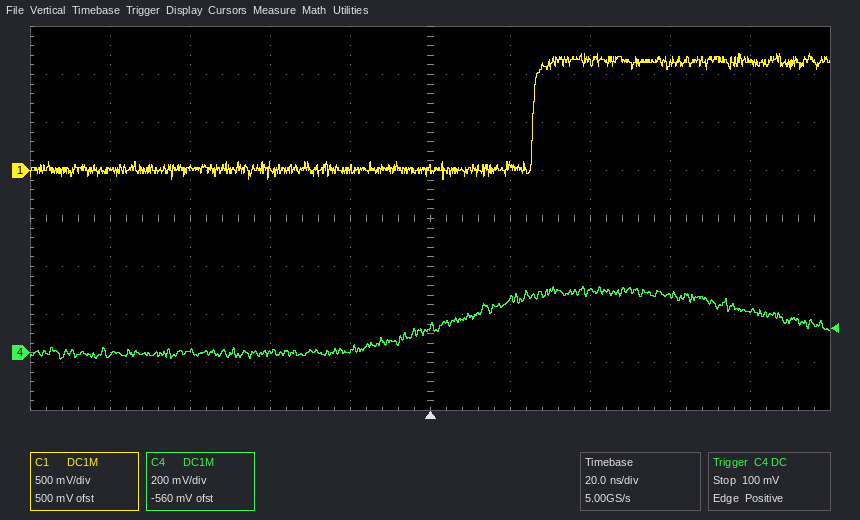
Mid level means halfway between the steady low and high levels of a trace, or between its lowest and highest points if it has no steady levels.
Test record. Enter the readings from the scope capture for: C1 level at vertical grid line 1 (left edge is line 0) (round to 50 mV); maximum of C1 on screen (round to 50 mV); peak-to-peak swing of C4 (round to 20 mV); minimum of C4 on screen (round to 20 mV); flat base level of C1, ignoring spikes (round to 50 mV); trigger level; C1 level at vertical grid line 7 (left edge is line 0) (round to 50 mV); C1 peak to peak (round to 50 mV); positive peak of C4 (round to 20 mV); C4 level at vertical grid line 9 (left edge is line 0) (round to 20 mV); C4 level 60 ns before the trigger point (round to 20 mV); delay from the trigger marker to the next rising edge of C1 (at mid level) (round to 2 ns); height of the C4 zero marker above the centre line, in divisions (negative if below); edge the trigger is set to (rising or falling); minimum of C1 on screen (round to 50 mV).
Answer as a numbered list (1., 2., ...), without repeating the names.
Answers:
1. 0 mV
2. 1.20 V
3. 300 mV
4. -20 mV
5. 0 mV
6. 100 mV
7. 1.15 V
8. 1.30 V
9. 280 mV
10. 180 mV
11. 0 mV
12. 26 ns
13. -2.8 div
14. rising
15. -100 mV
